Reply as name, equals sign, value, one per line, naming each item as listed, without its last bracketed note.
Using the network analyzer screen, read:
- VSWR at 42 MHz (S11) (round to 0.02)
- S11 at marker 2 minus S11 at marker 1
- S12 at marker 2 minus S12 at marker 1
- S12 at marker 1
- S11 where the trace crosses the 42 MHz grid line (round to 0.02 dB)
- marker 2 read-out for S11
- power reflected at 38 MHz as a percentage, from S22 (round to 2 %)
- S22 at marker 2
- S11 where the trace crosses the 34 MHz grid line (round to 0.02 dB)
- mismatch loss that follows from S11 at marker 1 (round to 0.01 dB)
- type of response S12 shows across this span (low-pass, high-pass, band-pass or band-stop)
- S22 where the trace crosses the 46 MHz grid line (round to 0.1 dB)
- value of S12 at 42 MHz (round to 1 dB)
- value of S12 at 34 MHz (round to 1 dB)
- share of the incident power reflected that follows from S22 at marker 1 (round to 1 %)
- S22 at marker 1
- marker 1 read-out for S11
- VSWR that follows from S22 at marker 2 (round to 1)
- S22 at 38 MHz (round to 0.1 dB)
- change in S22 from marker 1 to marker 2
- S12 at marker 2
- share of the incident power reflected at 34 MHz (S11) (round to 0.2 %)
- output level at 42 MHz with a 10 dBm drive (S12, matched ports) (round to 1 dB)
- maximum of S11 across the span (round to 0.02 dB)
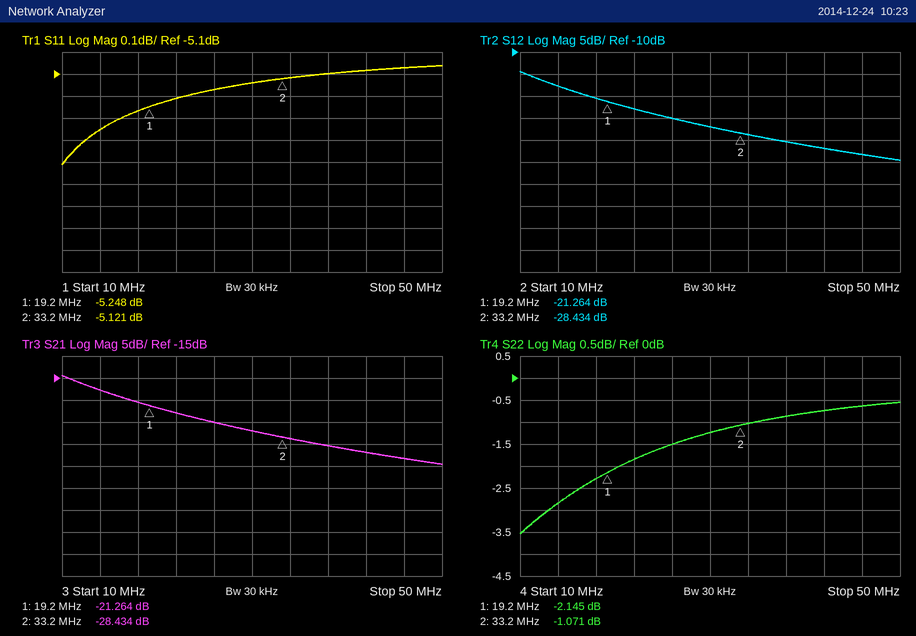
VSWR at 42 MHz (S11) = 3.52
S11 at marker 2 minus S11 at marker 1 = 0.127 dB
S12 at marker 2 minus S12 at marker 1 = -7.170 dB
S12 at marker 1 = -21.264 dB
S11 where the trace crosses the 42 MHz grid line = -5.08 dB
marker 2 read-out for S11 = -5.121 dB
power reflected at 38 MHz as a percentage, from S22 = 82 %
S22 at marker 2 = -1.071 dB
S11 where the trace crosses the 34 MHz grid line = -5.12 dB
mismatch loss that follows from S11 at marker 1 = 1.54 dB
type of response S12 shows across this span = low-pass
S22 where the trace crosses the 46 MHz grid line = -0.6 dB
value of S12 at 42 MHz = -32 dB
value of S12 at 34 MHz = -29 dB
share of the incident power reflected that follows from S22 at marker 1 = 61 %
S22 at marker 1 = -2.145 dB
marker 1 read-out for S11 = -5.248 dB
VSWR that follows from S22 at marker 2 = 16
S22 at 38 MHz = -0.9 dB
change in S22 from marker 1 to marker 2 = 1.074 dB
S12 at marker 2 = -28.434 dB
share of the incident power reflected at 34 MHz (S11) = 30.8 %
output level at 42 MHz with a 10 dBm drive (S12, matched ports) = -22 dBm
maximum of S11 across the span = -5.06 dB
